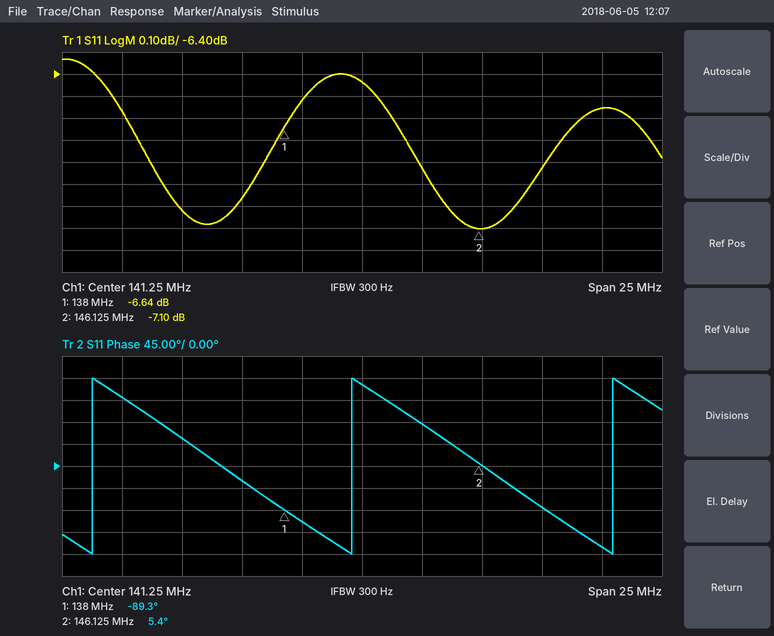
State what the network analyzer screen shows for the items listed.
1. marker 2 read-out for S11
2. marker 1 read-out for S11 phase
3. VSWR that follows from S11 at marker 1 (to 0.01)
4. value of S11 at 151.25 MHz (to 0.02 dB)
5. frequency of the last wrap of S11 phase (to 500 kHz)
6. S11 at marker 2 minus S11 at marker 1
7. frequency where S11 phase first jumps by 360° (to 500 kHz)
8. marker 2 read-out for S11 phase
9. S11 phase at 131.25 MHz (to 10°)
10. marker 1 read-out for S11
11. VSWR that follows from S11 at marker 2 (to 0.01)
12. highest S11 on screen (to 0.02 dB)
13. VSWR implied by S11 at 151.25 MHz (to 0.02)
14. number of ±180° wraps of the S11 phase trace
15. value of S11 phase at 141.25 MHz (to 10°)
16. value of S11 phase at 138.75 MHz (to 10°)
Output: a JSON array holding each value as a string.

["-7.10 dB", "-89.3°", "2.74", "-6.56 dB", "151.5 MHz", "-0.46 dB", "130.0 MHz", "5.4°", "140°", "-6.64 dB", "2.58", "-6.34 dB", "2.78", "3", "170°", "-110°"]
